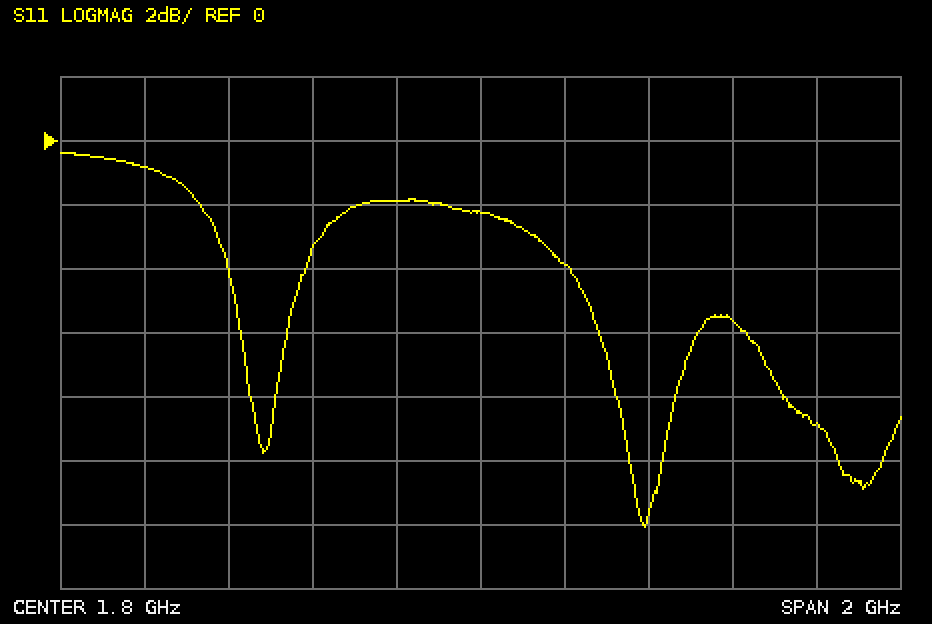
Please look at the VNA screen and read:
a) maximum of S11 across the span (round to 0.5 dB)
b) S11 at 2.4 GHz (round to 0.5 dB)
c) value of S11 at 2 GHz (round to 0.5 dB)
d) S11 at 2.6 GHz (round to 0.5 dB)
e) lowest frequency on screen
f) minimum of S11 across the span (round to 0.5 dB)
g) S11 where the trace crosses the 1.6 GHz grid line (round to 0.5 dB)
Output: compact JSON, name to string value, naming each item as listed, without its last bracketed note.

{"maximum of S11 across the span": "-0.5 dB", "S11 at 2.4 GHz": "-5.5 dB", "value of S11 at 2 GHz": "-4.0 dB", "S11 at 2.6 GHz": "-9.0 dB", "lowest frequency on screen": "800 MHz", "minimum of S11 across the span": "-12.0 dB", "S11 where the trace crosses the 1.6 GHz grid line": "-2.0 dB"}
